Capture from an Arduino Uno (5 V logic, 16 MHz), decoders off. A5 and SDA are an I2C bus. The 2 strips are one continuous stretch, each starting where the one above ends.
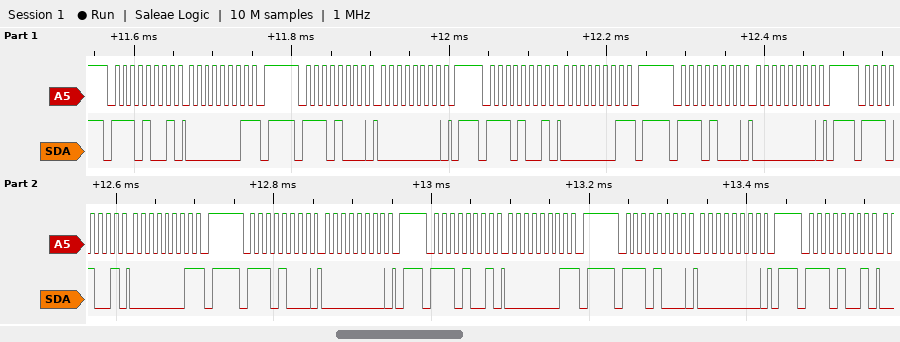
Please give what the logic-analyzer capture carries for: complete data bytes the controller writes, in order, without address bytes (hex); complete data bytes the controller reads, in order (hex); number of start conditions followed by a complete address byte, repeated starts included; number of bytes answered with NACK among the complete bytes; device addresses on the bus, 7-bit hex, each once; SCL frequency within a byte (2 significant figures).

00 00 00 00
01 01 01 01
9
4
0x74
100 kHz
